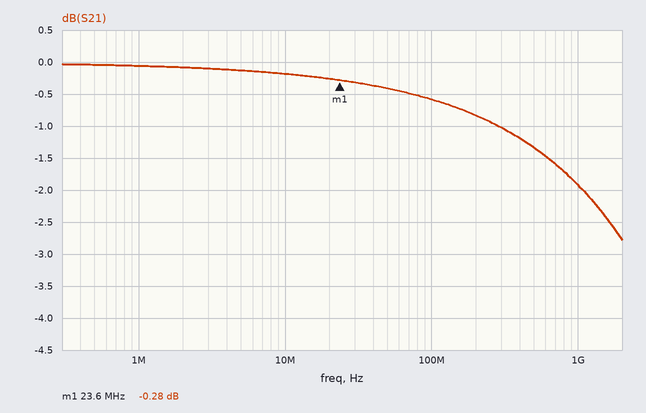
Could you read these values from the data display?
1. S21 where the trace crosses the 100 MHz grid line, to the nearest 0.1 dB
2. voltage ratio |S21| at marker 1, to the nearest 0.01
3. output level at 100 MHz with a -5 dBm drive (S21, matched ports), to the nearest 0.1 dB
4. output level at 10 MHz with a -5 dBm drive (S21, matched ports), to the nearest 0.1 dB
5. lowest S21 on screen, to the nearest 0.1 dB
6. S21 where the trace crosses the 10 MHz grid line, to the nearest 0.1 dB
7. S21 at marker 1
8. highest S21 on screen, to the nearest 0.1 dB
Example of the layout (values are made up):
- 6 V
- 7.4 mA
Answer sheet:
- -0.6 dB
- 0.97
- -5.6 dBm
- -5.2 dBm
- -2.8 dB
- -0.2 dB
- -0.28 dB
- 0.0 dB
